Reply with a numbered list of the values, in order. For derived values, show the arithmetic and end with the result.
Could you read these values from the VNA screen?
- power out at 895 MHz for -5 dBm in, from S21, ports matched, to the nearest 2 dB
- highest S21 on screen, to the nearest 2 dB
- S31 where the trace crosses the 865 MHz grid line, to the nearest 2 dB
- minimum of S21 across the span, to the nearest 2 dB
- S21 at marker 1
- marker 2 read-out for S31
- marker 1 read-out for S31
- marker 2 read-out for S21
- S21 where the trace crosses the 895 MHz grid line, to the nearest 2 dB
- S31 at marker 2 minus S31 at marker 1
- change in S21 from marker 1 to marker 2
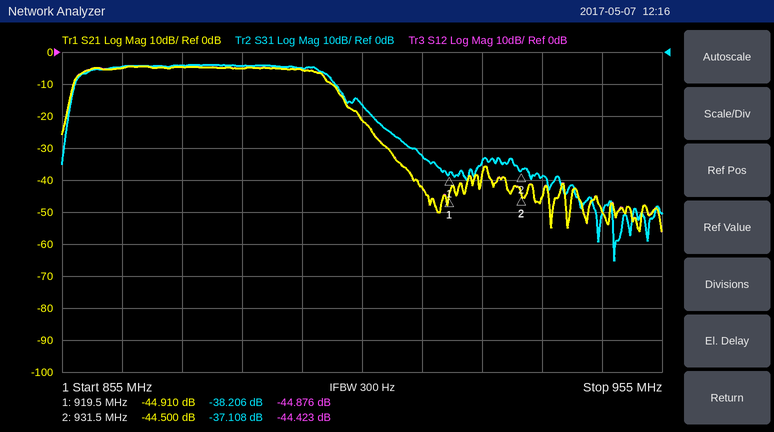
1. -5 dBm + (-6 dB) = -10 dBm
2. -4 dB
3. -4 dB
4. -56 dB
5. -44.910 dB
6. -37.108 dB
7. -38.206 dB
8. -44.500 dB
9. -6 dB
10. -37.108 − (-38.206) = 1.098 dB
11. -44.5 − (-44.91) = 0.410 dB
